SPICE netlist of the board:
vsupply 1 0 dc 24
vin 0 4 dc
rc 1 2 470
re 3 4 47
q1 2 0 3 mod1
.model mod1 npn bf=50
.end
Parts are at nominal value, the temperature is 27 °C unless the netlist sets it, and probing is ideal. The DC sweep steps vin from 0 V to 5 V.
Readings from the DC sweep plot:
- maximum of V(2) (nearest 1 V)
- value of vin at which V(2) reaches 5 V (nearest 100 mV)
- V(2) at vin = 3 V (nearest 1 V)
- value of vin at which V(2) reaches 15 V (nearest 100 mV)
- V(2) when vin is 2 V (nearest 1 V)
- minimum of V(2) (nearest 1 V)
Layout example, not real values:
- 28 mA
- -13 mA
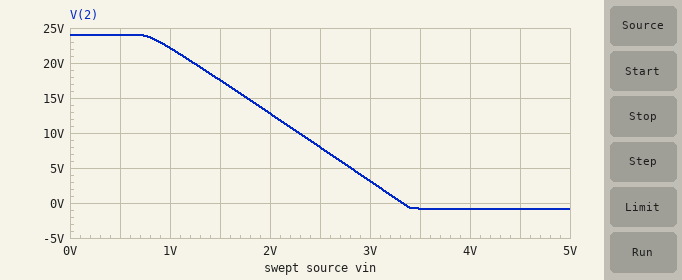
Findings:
- 24 V
- 2.8 V
- 3 V
- 1.8 V
- 13 V
- -1 V
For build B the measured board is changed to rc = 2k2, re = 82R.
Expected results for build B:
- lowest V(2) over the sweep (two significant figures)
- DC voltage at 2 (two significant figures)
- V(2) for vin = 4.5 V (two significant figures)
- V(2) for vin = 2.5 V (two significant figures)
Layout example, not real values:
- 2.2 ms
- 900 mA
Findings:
- -870 mV
- 24 V
- -860 mV
- -830 mV
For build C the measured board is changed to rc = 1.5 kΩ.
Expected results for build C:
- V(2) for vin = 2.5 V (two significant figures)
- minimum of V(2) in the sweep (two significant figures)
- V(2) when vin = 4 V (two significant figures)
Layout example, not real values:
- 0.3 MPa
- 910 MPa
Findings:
- -850 mV
- -880 mV
- -870 mV
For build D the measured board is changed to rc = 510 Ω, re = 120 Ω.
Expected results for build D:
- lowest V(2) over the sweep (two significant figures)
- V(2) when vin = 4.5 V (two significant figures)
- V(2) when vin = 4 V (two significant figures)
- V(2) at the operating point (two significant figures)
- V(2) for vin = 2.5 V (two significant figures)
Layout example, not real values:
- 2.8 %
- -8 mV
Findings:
- 6.8 V
- 8.8 V
- 11 V
- 24 V
- 17 V
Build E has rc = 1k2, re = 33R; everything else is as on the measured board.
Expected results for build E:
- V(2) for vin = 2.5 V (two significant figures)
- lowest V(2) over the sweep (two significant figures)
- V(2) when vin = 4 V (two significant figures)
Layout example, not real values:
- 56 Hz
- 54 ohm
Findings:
- -860 mV
- -890 mV
- -880 mV
